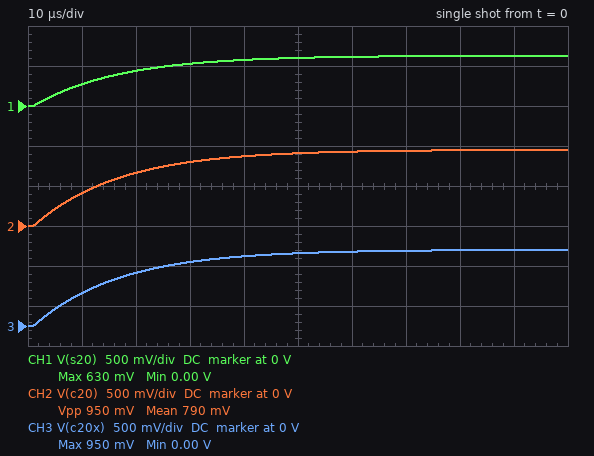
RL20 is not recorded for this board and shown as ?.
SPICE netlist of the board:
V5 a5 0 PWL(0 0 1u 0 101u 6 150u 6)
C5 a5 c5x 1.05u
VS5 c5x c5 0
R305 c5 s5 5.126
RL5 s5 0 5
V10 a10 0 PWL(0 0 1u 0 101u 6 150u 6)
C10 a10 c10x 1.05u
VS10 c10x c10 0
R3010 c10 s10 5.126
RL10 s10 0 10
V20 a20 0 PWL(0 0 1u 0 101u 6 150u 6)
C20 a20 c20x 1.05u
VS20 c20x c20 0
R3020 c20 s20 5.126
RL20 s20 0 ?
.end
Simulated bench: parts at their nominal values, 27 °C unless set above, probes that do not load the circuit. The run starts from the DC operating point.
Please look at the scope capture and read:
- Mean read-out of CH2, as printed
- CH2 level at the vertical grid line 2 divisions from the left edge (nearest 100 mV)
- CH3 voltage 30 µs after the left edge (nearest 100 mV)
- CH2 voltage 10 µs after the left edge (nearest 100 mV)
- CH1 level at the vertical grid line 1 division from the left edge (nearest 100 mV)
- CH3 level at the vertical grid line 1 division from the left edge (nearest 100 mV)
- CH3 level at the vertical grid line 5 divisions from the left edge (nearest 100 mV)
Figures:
790 mV
700 mV
800 mV
400 mV
300 mV
400 mV
900 mV
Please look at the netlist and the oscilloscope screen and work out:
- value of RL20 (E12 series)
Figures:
10 Ω
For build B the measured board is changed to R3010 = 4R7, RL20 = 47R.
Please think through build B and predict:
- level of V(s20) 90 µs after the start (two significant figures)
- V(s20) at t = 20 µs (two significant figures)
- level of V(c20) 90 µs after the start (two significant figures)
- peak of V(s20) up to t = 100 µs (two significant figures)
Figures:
2.4 V
870 mV
2.6 V
2.5 V
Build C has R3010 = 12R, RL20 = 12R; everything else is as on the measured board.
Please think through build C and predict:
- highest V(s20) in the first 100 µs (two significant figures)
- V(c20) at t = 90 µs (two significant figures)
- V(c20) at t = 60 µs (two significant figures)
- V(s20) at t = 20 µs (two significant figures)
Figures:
750 mV
1.1 V
1.0 V
490 mV
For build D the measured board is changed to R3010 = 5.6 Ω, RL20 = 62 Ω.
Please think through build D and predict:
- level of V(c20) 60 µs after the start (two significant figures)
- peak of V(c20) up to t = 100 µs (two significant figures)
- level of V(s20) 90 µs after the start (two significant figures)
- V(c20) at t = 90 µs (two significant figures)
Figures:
2.4 V
3.2 V
2.8 V
3.0 V
